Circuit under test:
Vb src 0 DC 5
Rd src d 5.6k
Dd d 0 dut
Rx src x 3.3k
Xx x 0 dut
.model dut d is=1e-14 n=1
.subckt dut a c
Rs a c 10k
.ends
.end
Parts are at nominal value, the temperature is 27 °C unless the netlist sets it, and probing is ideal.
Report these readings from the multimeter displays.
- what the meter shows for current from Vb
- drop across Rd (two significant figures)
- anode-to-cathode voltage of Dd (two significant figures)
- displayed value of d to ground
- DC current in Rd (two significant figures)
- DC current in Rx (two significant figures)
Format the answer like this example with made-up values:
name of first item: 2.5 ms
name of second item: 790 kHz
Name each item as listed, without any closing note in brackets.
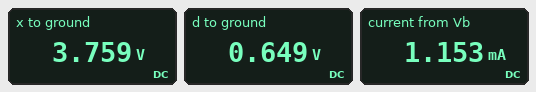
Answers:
what the meter shows for current from Vb: 1.153 mA
drop across Rd: 4.4 V
anode-to-cathode voltage of Dd: 650 mV
displayed value of d to ground: 0.649 V
DC current in Rd: 780 µA
DC current in Rx: 380 µA
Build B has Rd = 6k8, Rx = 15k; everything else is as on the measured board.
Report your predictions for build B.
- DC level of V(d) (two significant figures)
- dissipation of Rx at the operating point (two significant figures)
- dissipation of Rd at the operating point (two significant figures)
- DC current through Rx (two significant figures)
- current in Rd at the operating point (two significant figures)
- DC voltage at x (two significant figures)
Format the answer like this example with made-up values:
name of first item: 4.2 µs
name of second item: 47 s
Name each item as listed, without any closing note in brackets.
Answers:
DC level of V(d): 640 mV
dissipation of Rx at the operating point: 600 µW
dissipation of Rd at the operating point: 2.8 mW
DC current through Rx: 200 µA
current in Rd at the operating point: 640 µA
DC voltage at x: 2.0 V
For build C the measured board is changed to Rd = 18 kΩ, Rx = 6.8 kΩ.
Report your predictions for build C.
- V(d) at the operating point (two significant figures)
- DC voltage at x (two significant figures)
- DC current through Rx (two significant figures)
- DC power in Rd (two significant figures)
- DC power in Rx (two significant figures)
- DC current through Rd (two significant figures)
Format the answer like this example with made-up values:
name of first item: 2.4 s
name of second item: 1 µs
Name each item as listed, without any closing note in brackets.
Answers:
V(d) at the operating point: 620 mV
DC voltage at x: 3.0 V
DC current through Rx: 300 µA
DC power in Rd: 1.1 mW
DC power in Rx: 600 µW
DC current through Rd: 240 µA
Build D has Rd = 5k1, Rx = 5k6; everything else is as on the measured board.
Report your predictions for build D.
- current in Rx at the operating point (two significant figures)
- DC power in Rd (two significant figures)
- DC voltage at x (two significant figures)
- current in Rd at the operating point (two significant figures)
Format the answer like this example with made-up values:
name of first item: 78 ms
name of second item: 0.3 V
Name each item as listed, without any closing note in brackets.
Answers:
current in Rx at the operating point: 320 µA
DC power in Rd: 3.7 mW
DC voltage at x: 3.2 V
current in Rd at the operating point: 850 µA
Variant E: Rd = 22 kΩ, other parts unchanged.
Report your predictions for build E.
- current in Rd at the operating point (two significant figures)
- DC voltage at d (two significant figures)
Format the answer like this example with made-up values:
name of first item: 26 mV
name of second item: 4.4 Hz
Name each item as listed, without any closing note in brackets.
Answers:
current in Rd at the operating point: 200 µA
DC voltage at d: 610 mV
